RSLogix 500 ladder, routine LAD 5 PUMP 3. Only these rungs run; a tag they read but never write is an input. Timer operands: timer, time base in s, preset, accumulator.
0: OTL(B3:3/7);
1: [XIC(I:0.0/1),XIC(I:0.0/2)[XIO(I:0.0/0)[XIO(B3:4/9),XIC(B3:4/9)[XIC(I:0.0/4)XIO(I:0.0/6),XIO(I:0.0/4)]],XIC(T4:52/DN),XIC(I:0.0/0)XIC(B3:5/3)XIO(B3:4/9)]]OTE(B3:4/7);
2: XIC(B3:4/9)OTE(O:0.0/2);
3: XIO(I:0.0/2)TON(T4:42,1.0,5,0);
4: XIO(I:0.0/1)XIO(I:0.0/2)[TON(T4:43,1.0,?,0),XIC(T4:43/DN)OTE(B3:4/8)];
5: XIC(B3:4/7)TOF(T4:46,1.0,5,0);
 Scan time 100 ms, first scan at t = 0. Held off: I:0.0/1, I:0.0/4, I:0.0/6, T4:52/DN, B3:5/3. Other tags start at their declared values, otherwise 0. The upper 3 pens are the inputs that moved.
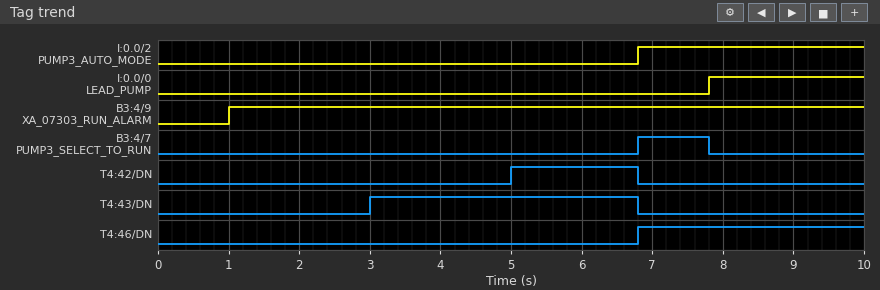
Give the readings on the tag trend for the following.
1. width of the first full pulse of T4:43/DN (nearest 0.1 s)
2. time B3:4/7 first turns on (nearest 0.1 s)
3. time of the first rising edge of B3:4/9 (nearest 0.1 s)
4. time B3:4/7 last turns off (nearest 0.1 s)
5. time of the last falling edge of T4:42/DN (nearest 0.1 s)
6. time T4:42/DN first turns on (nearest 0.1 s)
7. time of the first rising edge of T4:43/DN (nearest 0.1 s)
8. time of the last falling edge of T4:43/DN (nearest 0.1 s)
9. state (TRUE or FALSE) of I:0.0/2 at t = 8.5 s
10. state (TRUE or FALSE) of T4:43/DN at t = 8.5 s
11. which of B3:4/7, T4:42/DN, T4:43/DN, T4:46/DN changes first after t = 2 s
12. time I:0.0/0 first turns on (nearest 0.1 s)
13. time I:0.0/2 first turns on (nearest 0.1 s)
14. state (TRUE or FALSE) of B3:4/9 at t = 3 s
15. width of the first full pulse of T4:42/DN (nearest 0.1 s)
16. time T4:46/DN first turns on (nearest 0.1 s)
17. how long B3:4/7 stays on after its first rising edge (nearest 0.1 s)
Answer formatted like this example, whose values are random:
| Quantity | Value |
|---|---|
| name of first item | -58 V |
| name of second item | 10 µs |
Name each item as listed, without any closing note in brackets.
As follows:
| Quantity | Value |
|---|---|
| width of the first full pulse of T4:43/DN | 3.8 s |
| time B3:4/7 first turns on | 6.8 s |
| time of the first rising edge of B3:4/9 | 1.0 s |
| time B3:4/7 last turns off | 7.8 s |
| time of the last falling edge of T4:42/DN | 6.8 s |
| time T4:42/DN first turns on | 5.0 s |
| time of the first rising edge of T4:43/DN | 3.0 s |
| time of the last falling edge of T4:43/DN | 6.8 s |
| state (TRUE or FALSE) of I:0.0/2 at t = 8.5 s | TRUE |
| state (TRUE or FALSE) of T4:43/DN at t = 8.5 s | FALSE |
| which of B3:4/7, T4:42/DN, T4:43/DN, T4:46/DN changes first after t = 2 s | T4:43/DN |
| time I:0.0/0 first turns on | 7.8 s |
| time I:0.0/2 first turns on | 6.8 s |
| state (TRUE or FALSE) of B3:4/9 at t = 3 s | TRUE |
| width of the first full pulse of T4:42/DN | 1.8 s |
| time T4:46/DN first turns on | 6.8 s |
| how long B3:4/7 stays on after its first rising edge | 1.0 s |
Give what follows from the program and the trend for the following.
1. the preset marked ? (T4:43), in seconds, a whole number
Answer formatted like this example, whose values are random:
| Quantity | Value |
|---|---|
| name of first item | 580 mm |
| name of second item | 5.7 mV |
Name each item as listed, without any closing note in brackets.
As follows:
| Quantity | Value |
|---|---|
| the preset marked ? (T4:43), in seconds, a whole number | 3 s |
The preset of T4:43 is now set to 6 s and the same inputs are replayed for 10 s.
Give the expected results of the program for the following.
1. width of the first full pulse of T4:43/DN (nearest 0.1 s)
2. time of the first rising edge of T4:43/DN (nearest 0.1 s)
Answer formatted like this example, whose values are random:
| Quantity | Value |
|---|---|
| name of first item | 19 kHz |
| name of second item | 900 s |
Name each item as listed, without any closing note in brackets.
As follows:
| Quantity | Value |
|---|---|
| width of the first full pulse of T4:43/DN | 0.8 s |
| time of the first rising edge of T4:43/DN | 6.0 s |
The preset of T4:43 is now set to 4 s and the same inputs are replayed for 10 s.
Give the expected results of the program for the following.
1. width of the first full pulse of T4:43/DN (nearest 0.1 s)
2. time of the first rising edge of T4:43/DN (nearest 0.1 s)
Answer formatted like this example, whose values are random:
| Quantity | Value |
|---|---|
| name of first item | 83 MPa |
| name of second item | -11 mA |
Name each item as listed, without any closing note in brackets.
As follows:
| Quantity | Value |
|---|---|
| width of the first full pulse of T4:43/DN | 2.8 s |
| time of the first rising edge of T4:43/DN | 4.0 s |
